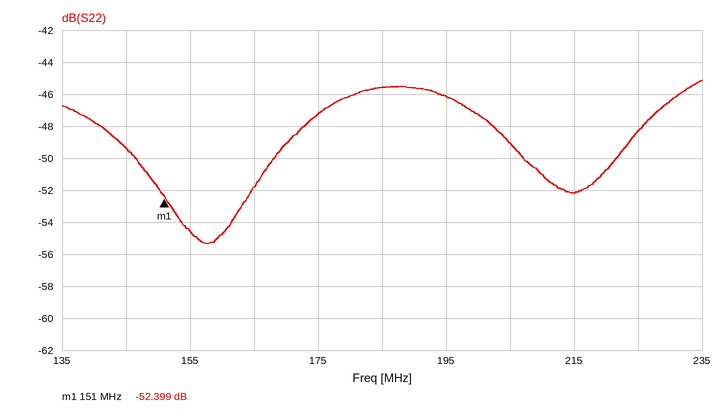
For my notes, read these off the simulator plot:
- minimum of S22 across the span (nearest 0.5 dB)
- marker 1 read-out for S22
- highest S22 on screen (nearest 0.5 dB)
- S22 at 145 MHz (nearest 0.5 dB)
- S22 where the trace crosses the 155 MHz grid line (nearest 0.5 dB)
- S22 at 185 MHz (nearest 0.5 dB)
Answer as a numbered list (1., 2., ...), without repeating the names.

1. -55.5 dB
2. -52.399 dB
3. -45.0 dB
4. -49.5 dB
5. -54.5 dB
6. -45.5 dB
